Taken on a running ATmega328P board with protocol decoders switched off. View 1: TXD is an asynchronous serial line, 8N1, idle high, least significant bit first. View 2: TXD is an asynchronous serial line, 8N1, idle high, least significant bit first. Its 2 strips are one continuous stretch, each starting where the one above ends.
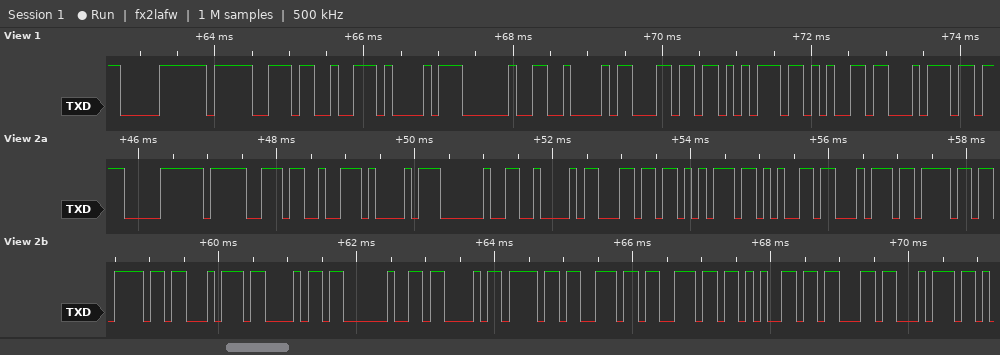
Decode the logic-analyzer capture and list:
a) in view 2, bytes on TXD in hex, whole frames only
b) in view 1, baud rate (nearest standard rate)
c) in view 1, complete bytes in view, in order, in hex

0xF0 0x9F 0x93 0xA1 0x20 0x42 0x6C 0x75 0x65 0x74 0x6F 0x6F 0x74 0x68 0x20 0x43 0x6F 0x6E 0x6E 0x65 0x63 0x74
9600 baud
F0 9F 93 A1 20 42 6C 75 65 74
